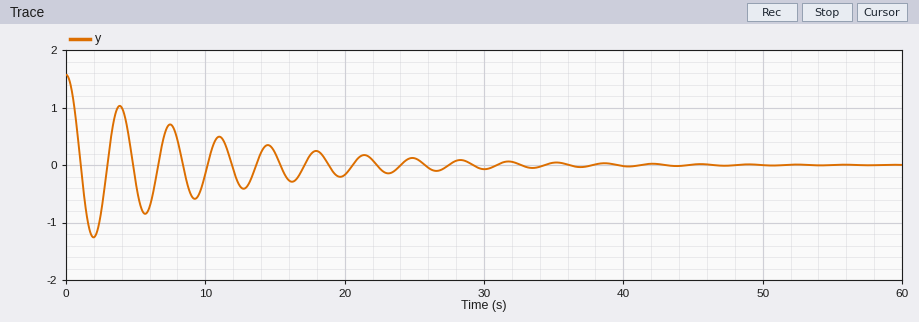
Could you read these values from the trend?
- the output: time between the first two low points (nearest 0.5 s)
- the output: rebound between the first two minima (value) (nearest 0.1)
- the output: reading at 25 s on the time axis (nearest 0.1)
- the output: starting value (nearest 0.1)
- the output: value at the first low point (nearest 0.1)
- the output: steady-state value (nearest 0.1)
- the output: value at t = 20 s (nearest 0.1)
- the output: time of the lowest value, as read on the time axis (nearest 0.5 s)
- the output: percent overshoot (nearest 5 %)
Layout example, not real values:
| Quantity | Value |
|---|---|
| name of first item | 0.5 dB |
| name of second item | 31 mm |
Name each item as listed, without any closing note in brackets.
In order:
| Quantity | Value |
|---|---|
| the output: time between the first two low points | 3.5 s |
| the output: rebound between the first two minima (value) | 1.0 |
| the output: reading at 25 s on the time axis | 0.1 |
| the output: starting value | 1.6 |
| the output: value at the first low point | -1.3 |
| the output: steady-state value | 0.0 |
| the output: value at t = 20 s | -0.2 |
| the output: time of the lowest value, as read on the time axis | 2.0 s |
| the output: percent overshoot | 80 % |
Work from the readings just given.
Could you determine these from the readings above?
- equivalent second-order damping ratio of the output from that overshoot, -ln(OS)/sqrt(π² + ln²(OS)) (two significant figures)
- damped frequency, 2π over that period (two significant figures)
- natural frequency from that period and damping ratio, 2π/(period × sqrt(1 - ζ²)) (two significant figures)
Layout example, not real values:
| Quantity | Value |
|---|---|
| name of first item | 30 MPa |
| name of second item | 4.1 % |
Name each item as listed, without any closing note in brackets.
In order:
| Quantity | Value |
|---|---|
| equivalent second-order damping ratio of the output from that overshoot, -ln(OS)/sqrt(π² + ln²(OS)) | 0.071 |
| damped frequency, 2π over that period | 1.8 rad/s |
| natural frequency from that period and damping ratio, 2π/(period × sqrt(1 - ζ²)) | 1.8 rad/s |
